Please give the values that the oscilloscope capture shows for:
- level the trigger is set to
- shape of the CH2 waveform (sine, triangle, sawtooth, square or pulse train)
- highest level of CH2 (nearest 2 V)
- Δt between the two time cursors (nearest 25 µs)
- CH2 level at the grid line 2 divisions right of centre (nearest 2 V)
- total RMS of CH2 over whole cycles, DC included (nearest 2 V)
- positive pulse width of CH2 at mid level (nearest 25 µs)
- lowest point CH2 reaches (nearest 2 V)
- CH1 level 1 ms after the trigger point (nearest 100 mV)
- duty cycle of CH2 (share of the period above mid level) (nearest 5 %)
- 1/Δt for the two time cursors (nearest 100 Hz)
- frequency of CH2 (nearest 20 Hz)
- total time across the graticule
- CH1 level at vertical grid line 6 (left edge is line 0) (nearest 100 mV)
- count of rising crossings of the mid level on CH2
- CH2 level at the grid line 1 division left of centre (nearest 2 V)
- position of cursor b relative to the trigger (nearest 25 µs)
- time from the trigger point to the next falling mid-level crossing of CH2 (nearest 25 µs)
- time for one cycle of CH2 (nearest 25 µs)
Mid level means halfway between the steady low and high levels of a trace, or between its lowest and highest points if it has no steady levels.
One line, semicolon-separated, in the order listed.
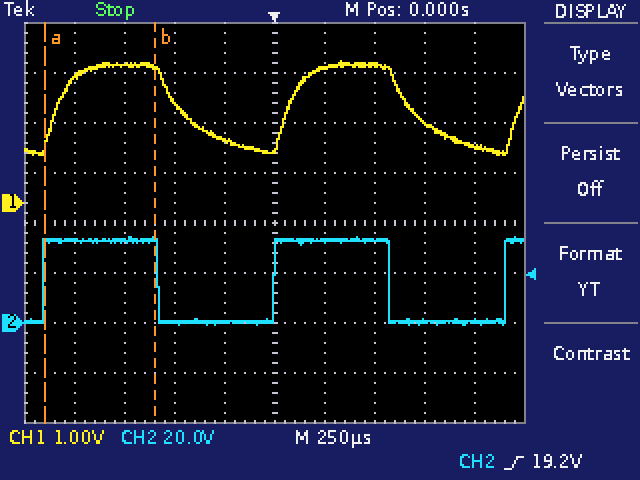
19.2 V; square; 34 V; 550 µs; 34 V; 24 V; 575 µs; 0 V; 1.1 V; 50 %; 1.8 kHz; 860 Hz; 2.5 ms; 2.7 V; 3; 0 V; -600 µs; 575 µs; 1.150 ms
